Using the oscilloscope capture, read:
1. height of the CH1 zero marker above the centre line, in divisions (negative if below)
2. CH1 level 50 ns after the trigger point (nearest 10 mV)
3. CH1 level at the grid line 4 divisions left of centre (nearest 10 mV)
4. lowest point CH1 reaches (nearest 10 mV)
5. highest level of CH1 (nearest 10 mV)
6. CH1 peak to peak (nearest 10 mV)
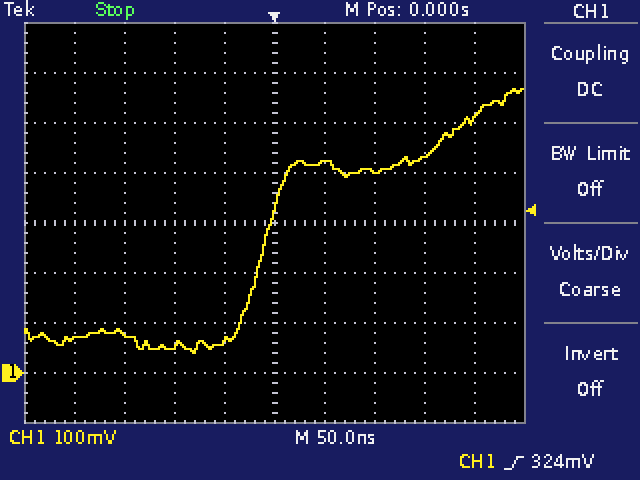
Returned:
-3.0 div
420 mV
70 mV
40 mV
570 mV
530 mV
